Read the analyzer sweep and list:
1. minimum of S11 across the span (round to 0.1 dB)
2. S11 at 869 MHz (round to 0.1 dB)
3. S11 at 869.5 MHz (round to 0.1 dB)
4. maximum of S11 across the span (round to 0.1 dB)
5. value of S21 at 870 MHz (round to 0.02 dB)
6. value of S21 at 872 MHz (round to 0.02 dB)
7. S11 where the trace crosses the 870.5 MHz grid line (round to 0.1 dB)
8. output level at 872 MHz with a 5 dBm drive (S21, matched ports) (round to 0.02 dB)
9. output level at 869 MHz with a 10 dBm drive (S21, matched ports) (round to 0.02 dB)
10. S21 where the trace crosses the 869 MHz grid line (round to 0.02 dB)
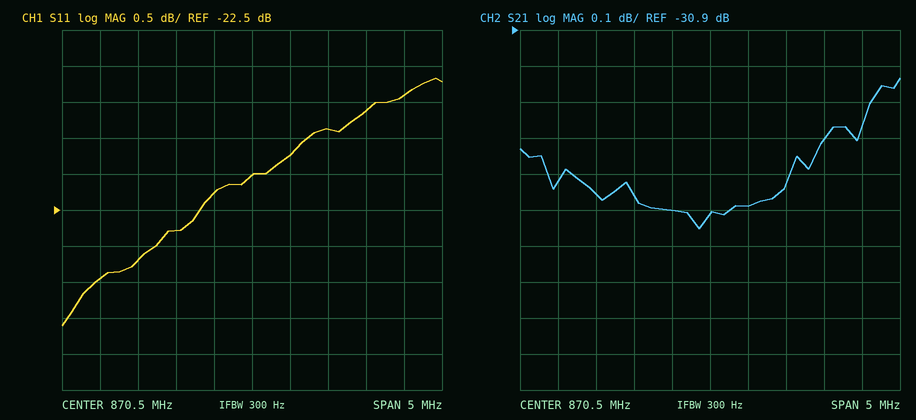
-24.1 dB
-23.2 dB
-22.8 dB
-20.7 dB
-31.40 dB
-31.20 dB
-22.0 dB
-26.20 dBm
-21.36 dBm
-31.36 dB
